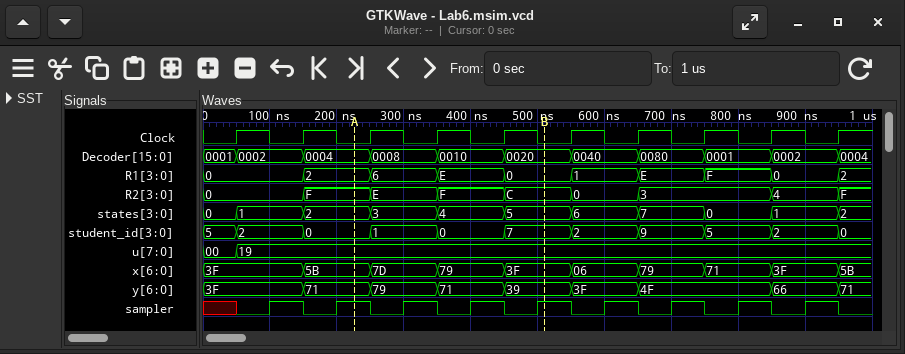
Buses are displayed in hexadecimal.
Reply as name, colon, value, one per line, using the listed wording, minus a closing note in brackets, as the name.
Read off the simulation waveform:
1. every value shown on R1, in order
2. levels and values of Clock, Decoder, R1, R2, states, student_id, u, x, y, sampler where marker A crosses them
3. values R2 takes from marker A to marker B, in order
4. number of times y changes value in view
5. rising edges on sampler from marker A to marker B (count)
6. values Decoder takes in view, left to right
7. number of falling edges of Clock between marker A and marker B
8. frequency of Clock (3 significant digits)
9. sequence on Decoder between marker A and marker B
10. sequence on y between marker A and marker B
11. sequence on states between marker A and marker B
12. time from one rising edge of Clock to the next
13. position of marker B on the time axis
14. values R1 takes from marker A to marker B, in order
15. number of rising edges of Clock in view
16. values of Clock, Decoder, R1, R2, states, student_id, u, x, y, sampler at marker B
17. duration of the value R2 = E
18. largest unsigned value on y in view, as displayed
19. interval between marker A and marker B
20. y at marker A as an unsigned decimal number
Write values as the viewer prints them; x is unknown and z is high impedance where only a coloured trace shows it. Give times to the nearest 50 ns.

every value shown on R1, in order: 0, 2, 6, E, 0, 1, E, F, 0, 2
levels and values of Clock, Decoder, R1, R2, states, student_id, u, x, y, sampler where marker A crosses them: Clock=0, Decoder=0004, R1=2, R2=F, states=2, student_id=0, u=19, x=5B, y=71, sampler=1
values R2 takes from marker A to marker B, in order: F, E, F, C
number of times y changes value in view: 8
rising edges on sampler from marker A to marker B: 3
values Decoder takes in view, left to right: 0001, 0002, 0004, 0008, 0010, 0020, 0040, 0080, 0001, 0002, 0004
number of falling edges of Clock between marker A and marker B: 3
frequency of Clock: 10.0 MHz
sequence on Decoder between marker A and marker B: 0004, 0008, 0010, 0020
sequence on y between marker A and marker B: 71, 79, 71, 39
sequence on states between marker A and marker B: 2, 3, 4, 5
time from one rising edge of Clock to the next: 100 ns
position of marker B on the time axis: 500 ns
values R1 takes from marker A to marker B, in order: 2, 6, E, 0
number of rising edges of Clock in view: 10
values of Clock, Decoder, R1, R2, states, student_id, u, x, y, sampler at marker B: Clock=0, Decoder=0020, R1=0, R2=C, states=5, student_id=7, u=19, x=3F, y=39, sampler=1
duration of the value R2 = E: 100 ns
largest unsigned value on y in view, as displayed: 79
interval between marker A and marker B: 300 ns
y at marker A as an unsigned decimal number: 113
